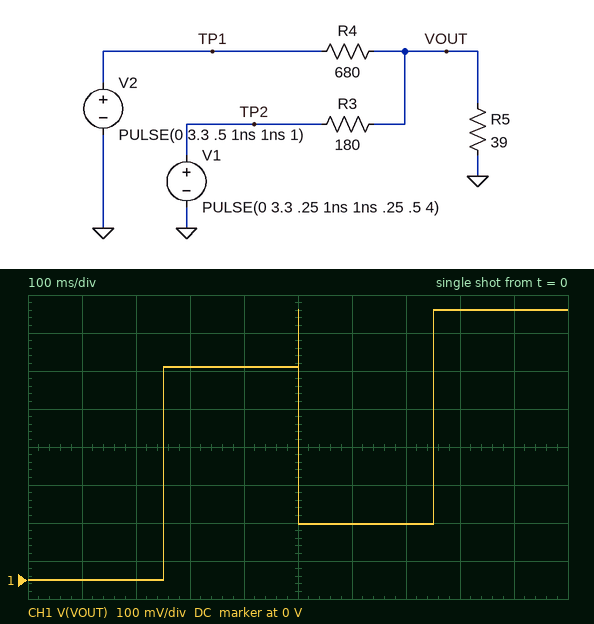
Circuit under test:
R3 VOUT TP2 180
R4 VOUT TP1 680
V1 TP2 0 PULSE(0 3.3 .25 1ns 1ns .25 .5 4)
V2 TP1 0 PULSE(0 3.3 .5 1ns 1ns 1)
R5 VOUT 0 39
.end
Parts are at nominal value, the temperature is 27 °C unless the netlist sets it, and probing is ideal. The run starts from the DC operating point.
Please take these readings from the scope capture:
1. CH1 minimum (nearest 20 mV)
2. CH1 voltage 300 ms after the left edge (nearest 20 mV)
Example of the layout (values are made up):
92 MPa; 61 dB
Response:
0 V; 560 mV
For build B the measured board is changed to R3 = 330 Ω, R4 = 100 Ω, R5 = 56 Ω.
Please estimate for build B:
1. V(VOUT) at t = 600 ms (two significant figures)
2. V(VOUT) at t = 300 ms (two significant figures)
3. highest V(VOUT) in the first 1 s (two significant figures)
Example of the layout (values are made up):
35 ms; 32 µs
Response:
1.1 V; 320 mV; 1.4 V
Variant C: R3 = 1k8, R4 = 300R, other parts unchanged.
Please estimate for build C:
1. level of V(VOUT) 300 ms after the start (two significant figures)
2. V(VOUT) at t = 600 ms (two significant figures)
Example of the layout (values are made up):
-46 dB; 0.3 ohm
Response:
62 mV; 370 mV
